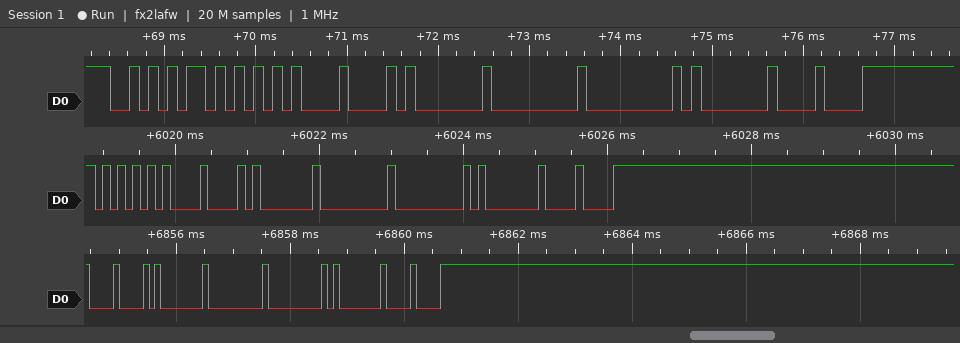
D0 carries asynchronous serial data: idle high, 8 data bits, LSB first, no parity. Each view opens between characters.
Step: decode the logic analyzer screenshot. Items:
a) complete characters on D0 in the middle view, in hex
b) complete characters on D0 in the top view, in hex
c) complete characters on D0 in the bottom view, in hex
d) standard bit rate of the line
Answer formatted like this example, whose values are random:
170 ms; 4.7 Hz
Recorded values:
55, 08, 01, 00, 00, 01, 08; AA, 55, 08, 01, 00, 00, 01, 08; 08, 01, 00, 00, 01, 08; 9600 baud
